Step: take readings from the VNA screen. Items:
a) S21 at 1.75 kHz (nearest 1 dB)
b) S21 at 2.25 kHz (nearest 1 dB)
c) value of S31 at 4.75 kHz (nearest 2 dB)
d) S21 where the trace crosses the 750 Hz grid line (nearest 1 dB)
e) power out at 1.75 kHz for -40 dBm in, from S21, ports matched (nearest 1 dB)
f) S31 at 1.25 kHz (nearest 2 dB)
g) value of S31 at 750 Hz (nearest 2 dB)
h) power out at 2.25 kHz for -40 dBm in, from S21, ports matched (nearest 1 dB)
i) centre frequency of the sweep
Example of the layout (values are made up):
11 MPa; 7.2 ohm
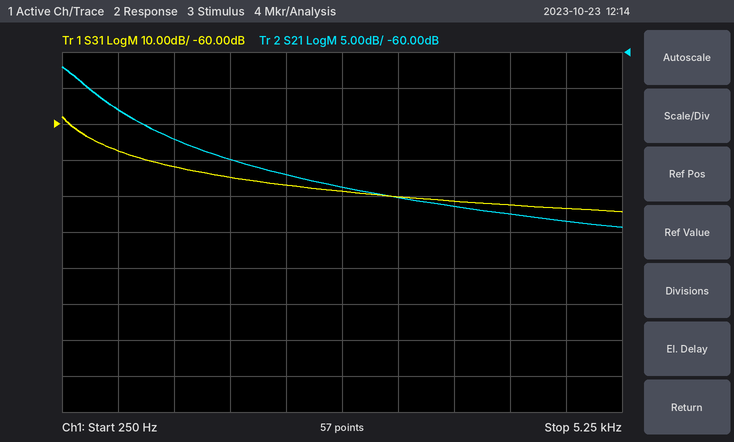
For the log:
-75 dB; -77 dB; -84 dB; -68 dB; -115 dBm; -72 dB; -68 dB; -117 dBm; 2.75 kHz
